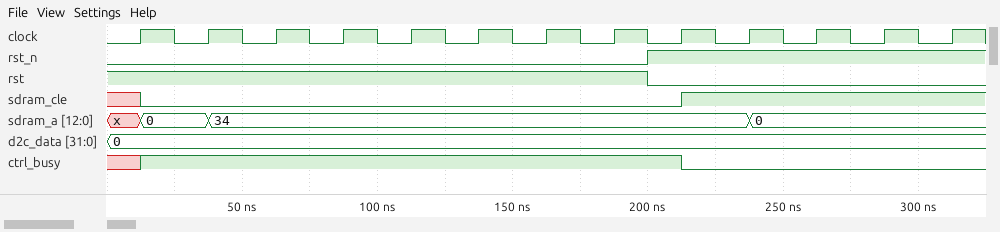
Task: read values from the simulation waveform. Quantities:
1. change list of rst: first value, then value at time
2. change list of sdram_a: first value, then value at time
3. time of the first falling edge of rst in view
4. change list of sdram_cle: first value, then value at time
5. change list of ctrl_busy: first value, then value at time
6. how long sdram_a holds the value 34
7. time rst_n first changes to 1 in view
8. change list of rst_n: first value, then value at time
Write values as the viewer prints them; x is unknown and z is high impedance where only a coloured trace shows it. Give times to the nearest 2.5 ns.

1, 0 at 200 ns
x, 0 at 12.5 ns, 34 at 37.5 ns, 0 at 237.5 ns
200 ns
x, 0 at 12.5 ns, 1 at 212.5 ns
x, 1 at 12.5 ns, 0 at 212.5 ns
200 ns
200 ns
0, 1 at 200 ns
